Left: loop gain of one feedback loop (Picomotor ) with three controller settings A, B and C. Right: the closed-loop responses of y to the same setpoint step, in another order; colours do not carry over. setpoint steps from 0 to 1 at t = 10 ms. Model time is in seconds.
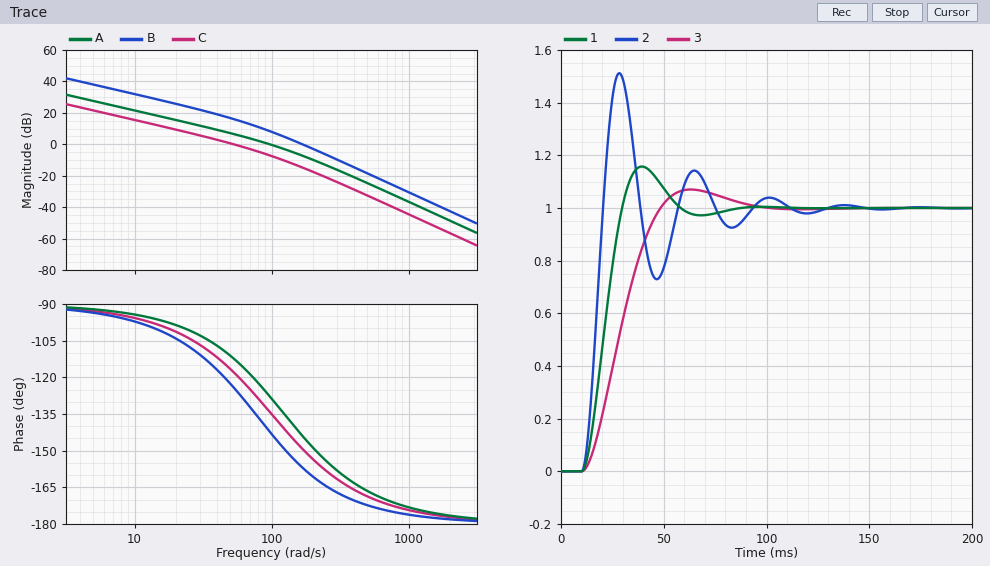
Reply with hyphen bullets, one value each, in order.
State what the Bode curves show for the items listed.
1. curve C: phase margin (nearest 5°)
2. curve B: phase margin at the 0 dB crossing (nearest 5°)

- 60°
- 25°
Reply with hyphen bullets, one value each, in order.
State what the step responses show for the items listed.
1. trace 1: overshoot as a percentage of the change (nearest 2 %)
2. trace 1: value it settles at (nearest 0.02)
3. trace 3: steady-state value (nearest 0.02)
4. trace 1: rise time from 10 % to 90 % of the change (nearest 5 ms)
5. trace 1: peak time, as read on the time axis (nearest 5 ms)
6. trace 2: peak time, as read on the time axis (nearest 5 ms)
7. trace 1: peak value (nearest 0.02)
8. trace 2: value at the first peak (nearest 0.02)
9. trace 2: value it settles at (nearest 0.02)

- 16 %
- 1.00
- 1.00
- 15 ms
- 40 ms
- 30 ms
- 1.16
- 1.52
- 1.00
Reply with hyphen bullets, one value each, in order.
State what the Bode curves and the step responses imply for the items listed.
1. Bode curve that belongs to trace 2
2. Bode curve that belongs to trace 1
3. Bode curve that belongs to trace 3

- B
- A
- C
